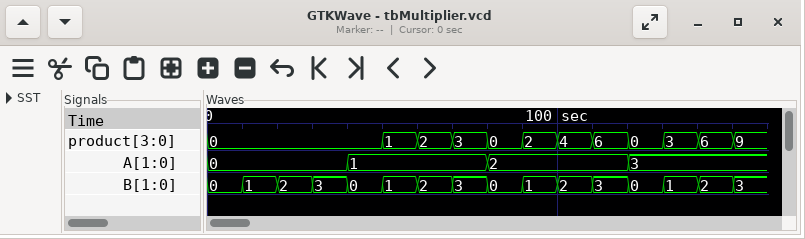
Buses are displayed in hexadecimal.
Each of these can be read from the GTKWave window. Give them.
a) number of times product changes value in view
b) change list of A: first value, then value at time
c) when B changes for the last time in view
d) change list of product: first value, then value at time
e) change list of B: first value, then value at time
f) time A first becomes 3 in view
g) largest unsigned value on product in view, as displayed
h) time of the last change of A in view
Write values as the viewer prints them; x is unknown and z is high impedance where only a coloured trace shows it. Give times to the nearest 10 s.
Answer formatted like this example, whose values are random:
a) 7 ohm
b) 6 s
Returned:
a) 11
b) 0, 1 at 40 s, 2 at 80 s, 3 at 120 s
c) 150 s
d) 0, 1 at 50 s, 2 at 60 s, 3 at 70 s, 0 at 80 s, 2 at 90 s, 4 at 100 s, 6 at 110 s, 0 at 120 s, 3 at 130 s, 6 at 140 s, 9 at 150 s
e) 0, 1 at 10 s, 2 at 20 s, 3 at 30 s, 0 at 40 s, 1 at 50 s, 2 at 60 s, 3 at 70 s, 0 at 80 s, 1 at 90 s, 2 at 100 s, 3 at 110 s, 0 at 120 s, 1 at 130 s, 2 at 140 s, 3 at 150 s
f) 120 s
g) 9
h) 120 s
